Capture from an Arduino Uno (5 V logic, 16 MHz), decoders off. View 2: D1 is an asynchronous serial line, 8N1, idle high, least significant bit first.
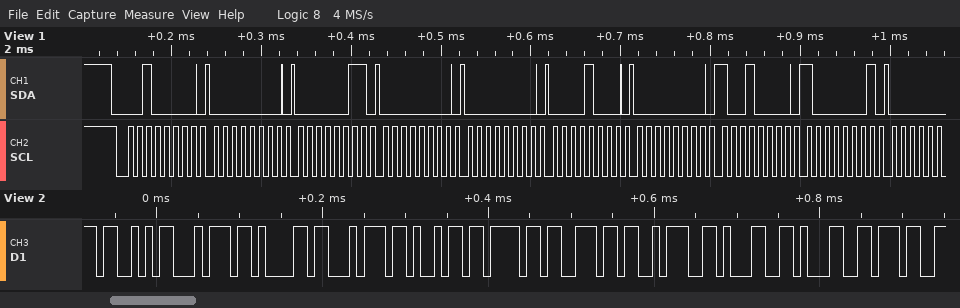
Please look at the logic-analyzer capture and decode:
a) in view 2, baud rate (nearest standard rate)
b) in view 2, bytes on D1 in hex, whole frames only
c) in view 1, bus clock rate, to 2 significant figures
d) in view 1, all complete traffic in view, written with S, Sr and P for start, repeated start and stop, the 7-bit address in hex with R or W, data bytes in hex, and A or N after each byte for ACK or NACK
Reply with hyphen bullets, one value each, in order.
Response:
- 115200 baud
- 0x53 0x74 0x61 0x74 0x69 0x6F 0x6E 0x3A 0x31 0x31 0x37
- 100 kHz
- S 10W A 00 A 03 A 00 A 00 A 08 A 00 A 90 A 81 A
